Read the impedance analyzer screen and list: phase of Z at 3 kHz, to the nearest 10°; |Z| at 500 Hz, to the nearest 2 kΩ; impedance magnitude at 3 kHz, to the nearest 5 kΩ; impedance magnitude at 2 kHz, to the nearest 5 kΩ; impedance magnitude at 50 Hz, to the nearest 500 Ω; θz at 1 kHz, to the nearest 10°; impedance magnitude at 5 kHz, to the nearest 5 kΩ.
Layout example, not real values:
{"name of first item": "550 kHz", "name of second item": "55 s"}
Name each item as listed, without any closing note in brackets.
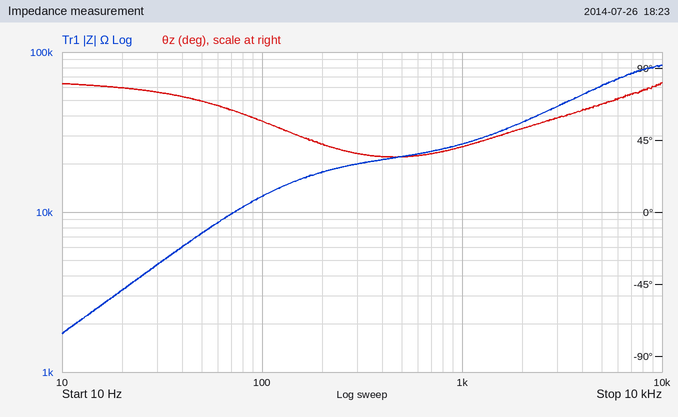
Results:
{"phase of Z at 3 kHz, to the nearest 10°": "60°", "|Z| at 500 Hz, to the nearest 2 kΩ": "22 kΩ", "impedance magnitude at 3 kHz, to the nearest 5 kΩ": "45 kΩ", "impedance magnitude at 2 kHz, to the nearest 5 kΩ": "35 kΩ", "impedance magnitude at 50 Hz, to the nearest 500 Ω": "7.5 kΩ", "θz at 1 kHz, to the nearest 10°": "40°", "impedance magnitude at 5 kHz, to the nearest 5 kΩ": "60 kΩ"}
